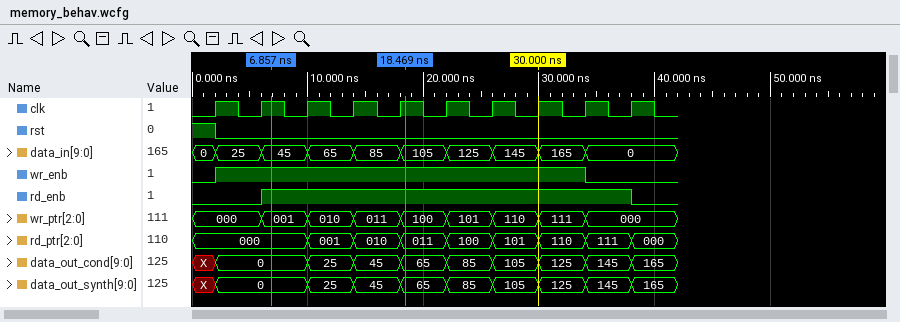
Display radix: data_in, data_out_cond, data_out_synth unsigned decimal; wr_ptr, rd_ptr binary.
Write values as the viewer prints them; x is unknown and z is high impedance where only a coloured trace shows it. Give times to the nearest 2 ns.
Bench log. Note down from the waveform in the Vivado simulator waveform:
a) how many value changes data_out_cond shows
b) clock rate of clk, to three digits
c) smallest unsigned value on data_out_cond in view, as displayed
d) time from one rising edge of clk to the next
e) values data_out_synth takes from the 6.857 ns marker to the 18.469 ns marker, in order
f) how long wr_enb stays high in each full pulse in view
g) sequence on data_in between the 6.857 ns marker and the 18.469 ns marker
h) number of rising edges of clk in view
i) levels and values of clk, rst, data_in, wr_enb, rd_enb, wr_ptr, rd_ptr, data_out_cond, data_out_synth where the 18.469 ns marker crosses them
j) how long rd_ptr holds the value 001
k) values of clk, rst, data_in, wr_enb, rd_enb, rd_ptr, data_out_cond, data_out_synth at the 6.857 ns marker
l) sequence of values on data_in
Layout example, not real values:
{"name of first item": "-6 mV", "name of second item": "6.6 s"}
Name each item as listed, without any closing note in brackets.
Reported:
{"how many value changes data_out_cond shows": "9", "clock rate of clk, to three digits": "250 MHz", "smallest unsigned value on data_out_cond in view, as displayed": "0", "time from one rising edge of clk to the next": "4 ns", "values data_out_synth takes from the 6.857 ns marker to the 18.469 ns marker, in order": "0, 25, 45, 65", "how long wr_enb stays high in each full pulse in view": "32 ns", "sequence on data_in between the 6.857 ns marker and the 18.469 ns marker": "45, 65, 85, 105", "number of rising edges of clk in view": "10", "levels and values of clk, rst, data_in, wr_enb, rd_enb, wr_ptr, rd_ptr, data_out_cond, data_out_synth where the 18.469 ns marker crosses them": "clk=1, rst=0, data_in=105, wr_enb=1, rd_enb=1, wr_ptr=100, rd_ptr=011, data_out_cond=65, data_out_synth=65", "how long rd_ptr holds the value 001": "4 ns", "values of clk, rst, data_in, wr_enb, rd_enb, rd_ptr, data_out_cond, data_out_synth at the 6.857 ns marker": "clk=1, rst=0, data_in=45, wr_enb=1, rd_enb=1, rd_ptr=000, data_out_cond=0, data_out_synth=0", "sequence of values on data_in": "0, 25, 45, 65, 85, 105, 125, 145, 165, 0"}
